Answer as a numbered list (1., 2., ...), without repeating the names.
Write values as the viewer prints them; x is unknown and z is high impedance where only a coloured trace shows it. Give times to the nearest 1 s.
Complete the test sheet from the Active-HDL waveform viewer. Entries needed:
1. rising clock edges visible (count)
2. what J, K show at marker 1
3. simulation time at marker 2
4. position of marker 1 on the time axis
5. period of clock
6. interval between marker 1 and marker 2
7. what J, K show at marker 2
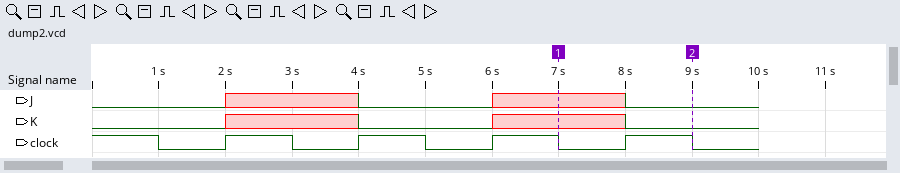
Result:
1. 4
2. J=x, K=x
3. 9 s
4. 7 s
5. 2 s
6. 2 s
7. J=0, K=0
